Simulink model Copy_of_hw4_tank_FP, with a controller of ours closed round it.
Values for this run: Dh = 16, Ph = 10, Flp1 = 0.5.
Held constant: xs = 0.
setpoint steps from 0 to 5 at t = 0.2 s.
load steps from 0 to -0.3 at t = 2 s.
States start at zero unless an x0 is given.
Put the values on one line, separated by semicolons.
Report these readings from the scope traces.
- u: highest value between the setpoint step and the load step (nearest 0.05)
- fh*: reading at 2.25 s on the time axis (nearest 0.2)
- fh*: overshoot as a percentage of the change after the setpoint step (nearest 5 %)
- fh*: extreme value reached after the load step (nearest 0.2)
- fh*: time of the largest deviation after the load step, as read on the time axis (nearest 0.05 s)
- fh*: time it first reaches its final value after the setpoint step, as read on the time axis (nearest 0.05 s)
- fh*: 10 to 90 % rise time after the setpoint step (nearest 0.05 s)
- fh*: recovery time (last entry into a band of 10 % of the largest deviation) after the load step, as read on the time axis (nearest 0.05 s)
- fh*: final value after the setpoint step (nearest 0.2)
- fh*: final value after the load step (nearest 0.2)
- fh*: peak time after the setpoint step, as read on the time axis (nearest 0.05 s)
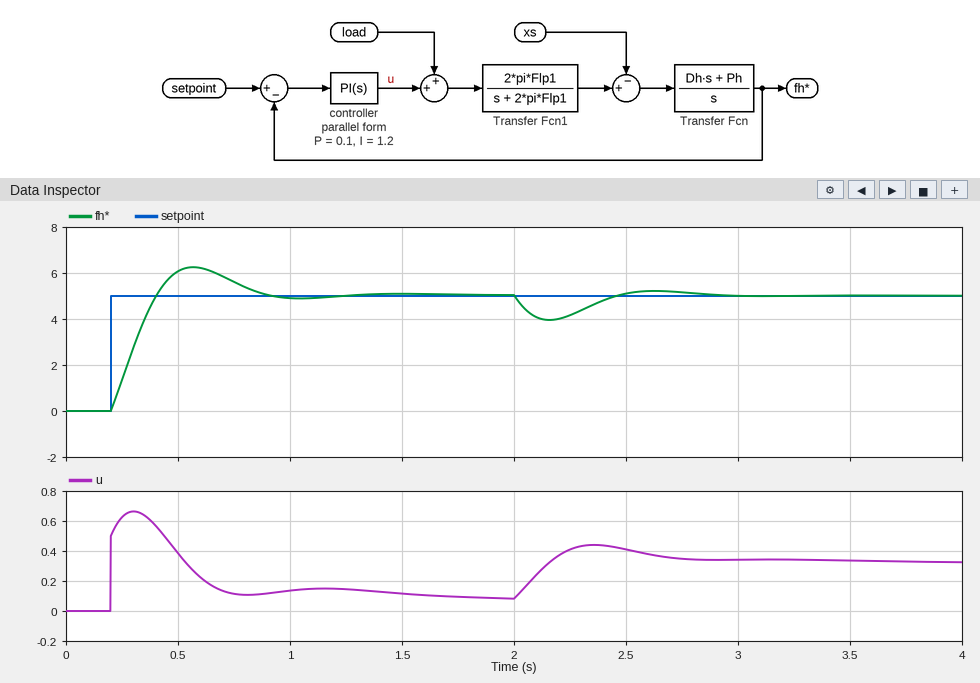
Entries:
0.65; 4.2; 25 %; 4.0; 2.15 s; 0.40 s; 0.15 s; 2.80 s; 5.0; 5.0; 0.55 s
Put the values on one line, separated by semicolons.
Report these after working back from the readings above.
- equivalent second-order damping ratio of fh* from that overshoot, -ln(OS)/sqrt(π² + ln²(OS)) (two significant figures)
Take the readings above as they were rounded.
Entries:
0.40
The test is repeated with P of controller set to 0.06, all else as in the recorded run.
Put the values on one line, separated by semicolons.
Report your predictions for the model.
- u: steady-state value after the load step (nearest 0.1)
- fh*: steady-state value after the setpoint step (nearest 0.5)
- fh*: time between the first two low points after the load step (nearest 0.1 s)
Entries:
0.3; 5.0; 0.9 s
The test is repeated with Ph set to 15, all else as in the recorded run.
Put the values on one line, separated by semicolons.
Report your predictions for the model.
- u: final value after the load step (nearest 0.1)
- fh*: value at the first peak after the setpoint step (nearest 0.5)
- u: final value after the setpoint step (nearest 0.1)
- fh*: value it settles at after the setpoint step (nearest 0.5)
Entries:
0.3; 6.5; 0.0; 5.0
